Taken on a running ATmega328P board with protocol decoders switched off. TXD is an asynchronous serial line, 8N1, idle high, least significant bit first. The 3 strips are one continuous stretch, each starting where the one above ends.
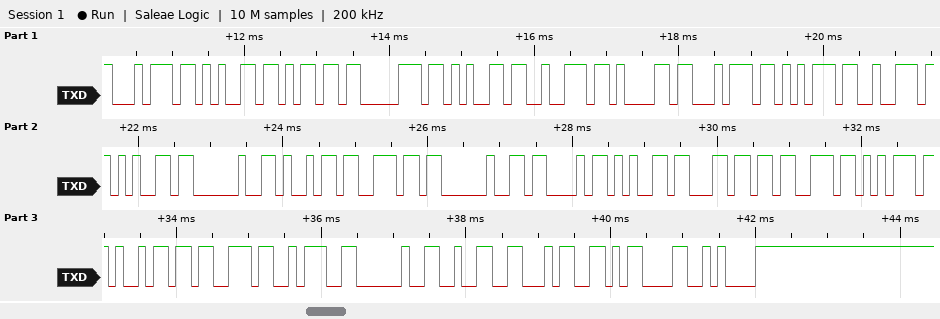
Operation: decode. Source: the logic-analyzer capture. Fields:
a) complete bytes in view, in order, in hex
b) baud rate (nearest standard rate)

74 65 6D 70 65 72 61 74 75 72 65 20 69 6E 20 43 65 6C 73 75 69 73 3A 20 32 34 0D 0A
9600 baud
